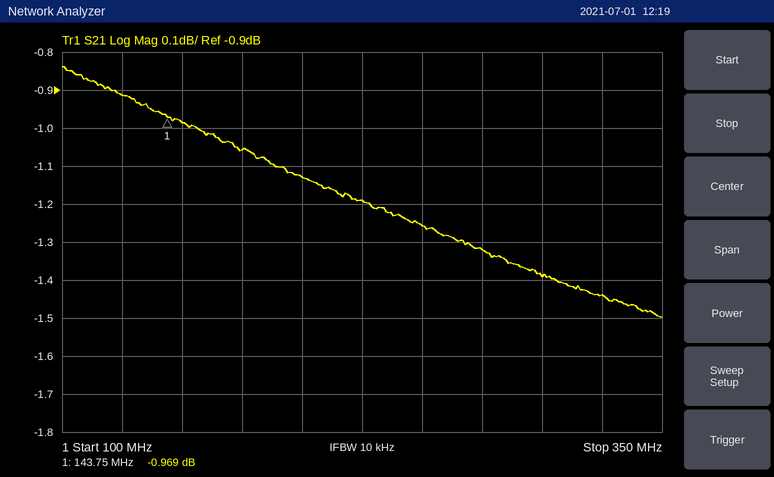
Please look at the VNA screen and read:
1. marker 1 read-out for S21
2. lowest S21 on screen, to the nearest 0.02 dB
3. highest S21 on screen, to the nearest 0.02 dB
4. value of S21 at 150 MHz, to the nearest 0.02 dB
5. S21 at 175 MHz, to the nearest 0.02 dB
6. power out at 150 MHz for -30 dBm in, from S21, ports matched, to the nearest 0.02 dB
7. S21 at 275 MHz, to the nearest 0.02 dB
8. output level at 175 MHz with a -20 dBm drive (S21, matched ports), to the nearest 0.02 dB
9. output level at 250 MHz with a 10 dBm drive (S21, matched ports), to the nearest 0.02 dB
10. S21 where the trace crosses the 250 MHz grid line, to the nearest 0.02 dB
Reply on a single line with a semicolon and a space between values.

-0.969 dB; -1.50 dB; -0.84 dB; -0.98 dB; -1.06 dB; -30.98 dBm; -1.32 dB; -21.06 dBm; 8.74 dBm; -1.26 dB
